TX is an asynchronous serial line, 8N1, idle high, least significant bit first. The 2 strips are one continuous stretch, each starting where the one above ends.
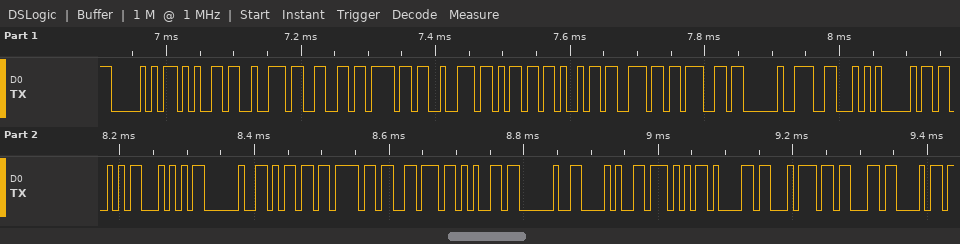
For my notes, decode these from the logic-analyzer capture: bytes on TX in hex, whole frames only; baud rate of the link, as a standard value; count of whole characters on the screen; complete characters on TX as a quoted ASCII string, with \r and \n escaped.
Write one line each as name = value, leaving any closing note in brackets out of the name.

bytes on TX in hex, whole frames only = 0x50 0x65 0x72 0x66 0x6F 0x72 0x6D 0x69 0x6E 0x67 0x20 0x46 0x41 0x53 0x54 0x20 0x6D 0x6F 0x76 0x65 0x20 0x28 0x57 0x61 0x74 0x63 0x68
baud rate of the link, as a standard value = 115200 baud
count of whole characters on the screen = 27
complete characters on TX as a quoted ASCII string, with \r and \n escaped = "Performing FAST move (Watch"
